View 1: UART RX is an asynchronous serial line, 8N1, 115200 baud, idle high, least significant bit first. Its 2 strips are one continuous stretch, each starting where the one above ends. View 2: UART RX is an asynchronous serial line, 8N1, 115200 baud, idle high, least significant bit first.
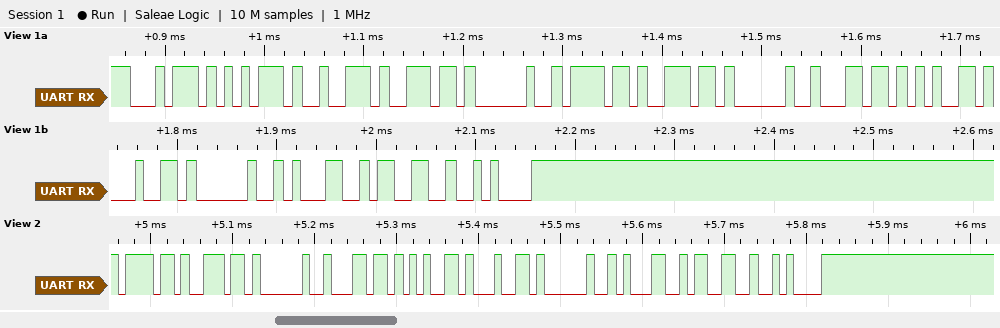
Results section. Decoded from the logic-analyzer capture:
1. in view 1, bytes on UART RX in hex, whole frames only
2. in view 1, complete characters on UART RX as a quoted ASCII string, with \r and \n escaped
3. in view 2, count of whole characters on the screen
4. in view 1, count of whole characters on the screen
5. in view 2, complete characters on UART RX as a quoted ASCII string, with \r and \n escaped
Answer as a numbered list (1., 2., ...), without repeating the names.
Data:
1. 74 75 72 6E 20 6F 6E 20 6C 65 64 20 31 33 0A
2. "turn on led 13\n"
3. 10
4. 15
5. "on led 13\n"
